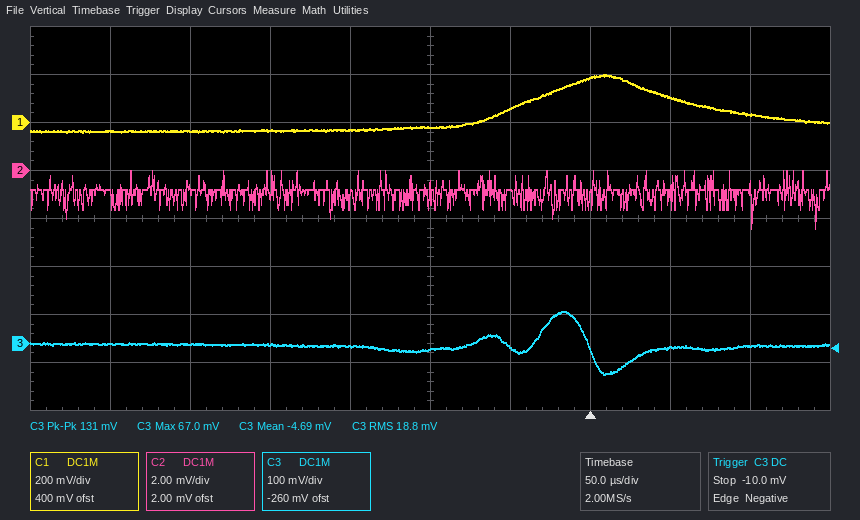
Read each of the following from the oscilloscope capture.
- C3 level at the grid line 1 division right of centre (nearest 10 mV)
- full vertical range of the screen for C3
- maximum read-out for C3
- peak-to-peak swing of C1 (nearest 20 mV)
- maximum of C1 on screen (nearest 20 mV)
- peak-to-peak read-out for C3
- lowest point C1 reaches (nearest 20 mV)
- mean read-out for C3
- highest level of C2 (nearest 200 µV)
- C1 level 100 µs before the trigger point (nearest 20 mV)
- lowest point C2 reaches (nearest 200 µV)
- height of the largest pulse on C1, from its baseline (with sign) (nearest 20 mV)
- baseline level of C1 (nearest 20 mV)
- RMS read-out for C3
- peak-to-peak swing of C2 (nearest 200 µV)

-10 mV
800 mV
67.0 mV
240 mV
200 mV
131 mV
-40 mV
-4.69 mV
0.0 mV
-20 mV
-2.4 mV
+240 mV
-40 mV
18.8 mV
2.4 mV
